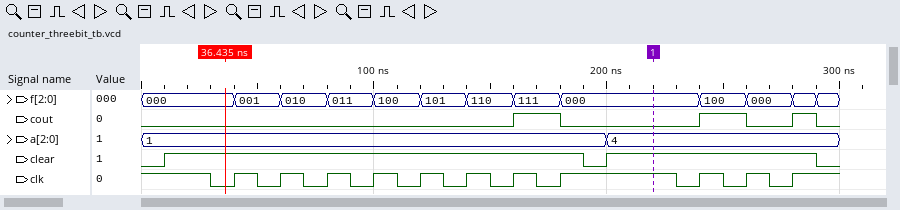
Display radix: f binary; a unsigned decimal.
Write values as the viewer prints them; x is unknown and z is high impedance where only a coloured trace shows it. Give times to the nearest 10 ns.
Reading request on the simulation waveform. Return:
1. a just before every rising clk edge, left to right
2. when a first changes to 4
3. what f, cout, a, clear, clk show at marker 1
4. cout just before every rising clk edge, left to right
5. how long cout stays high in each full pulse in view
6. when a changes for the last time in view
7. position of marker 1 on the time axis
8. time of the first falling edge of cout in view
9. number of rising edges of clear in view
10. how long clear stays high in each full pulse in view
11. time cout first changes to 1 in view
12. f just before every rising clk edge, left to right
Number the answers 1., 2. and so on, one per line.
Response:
1. 1, 1, 1, 1, 1, 1, 1, 1, 4, 4, 4
2. 200 ns
3. f=000, cout=0, a=4, clear=1, clk=1
4. 0 0 0 0 0 0 0 1 0 1 0
5. 20 ns, 20 ns, 10 ns
6. 200 ns
7. 220 ns
8. 180 ns
9. 2
10. 180 ns, 90 ns
11. 160 ns
12. 000, 001, 010, 011, 100, 101, 110, 111, 000, 100, 000
